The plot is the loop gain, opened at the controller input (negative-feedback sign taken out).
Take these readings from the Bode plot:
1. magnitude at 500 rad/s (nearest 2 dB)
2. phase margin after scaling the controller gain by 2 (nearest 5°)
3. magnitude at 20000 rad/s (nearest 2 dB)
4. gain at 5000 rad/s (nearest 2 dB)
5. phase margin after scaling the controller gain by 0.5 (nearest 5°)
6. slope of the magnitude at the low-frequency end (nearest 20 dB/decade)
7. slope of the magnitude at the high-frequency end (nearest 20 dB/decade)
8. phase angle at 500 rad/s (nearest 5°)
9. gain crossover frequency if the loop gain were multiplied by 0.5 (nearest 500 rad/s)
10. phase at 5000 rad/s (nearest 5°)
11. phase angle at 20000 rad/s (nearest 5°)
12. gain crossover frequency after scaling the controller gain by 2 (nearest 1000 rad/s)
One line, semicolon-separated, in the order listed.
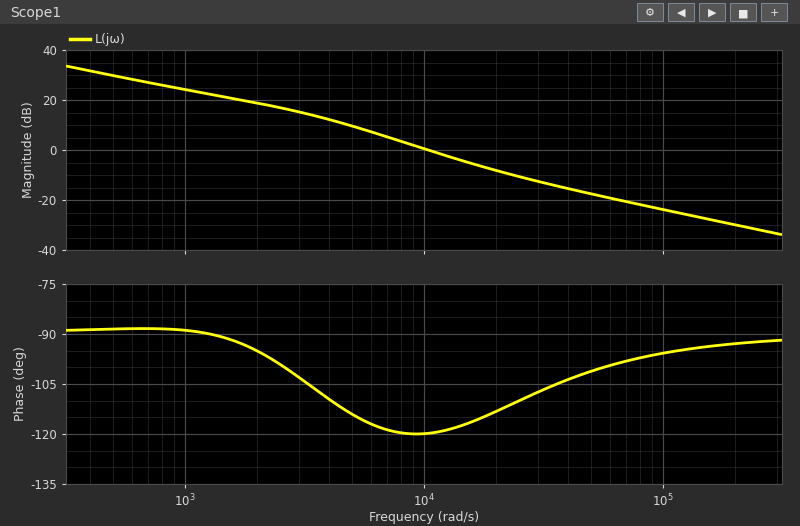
30 dB; 65°; -8 dB; 10 dB; 60°; -20 dB/decade; -20 dB/decade; -90°; 6500 rad/s; -115°; -115°; 17000 rad/s
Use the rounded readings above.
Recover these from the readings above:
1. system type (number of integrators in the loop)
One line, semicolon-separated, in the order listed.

1
